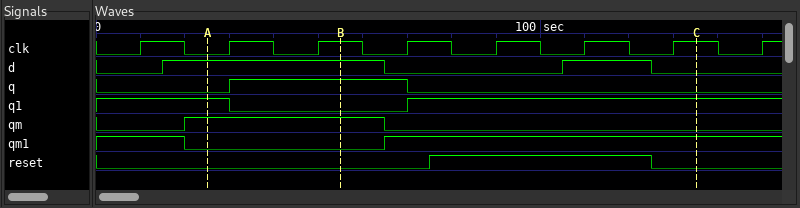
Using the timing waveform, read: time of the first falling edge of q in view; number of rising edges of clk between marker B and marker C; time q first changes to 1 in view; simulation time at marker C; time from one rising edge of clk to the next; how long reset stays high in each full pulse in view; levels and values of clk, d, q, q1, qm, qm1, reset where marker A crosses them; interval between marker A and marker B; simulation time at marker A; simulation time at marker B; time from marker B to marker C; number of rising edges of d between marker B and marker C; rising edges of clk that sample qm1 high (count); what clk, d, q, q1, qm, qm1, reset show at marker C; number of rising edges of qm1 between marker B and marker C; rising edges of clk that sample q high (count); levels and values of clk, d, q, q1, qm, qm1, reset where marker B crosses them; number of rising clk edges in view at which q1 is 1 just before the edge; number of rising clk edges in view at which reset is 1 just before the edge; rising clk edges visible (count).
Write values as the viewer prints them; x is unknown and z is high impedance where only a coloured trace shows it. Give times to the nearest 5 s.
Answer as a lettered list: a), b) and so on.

a) 70 s
b) 4
c) 30 s
d) 135 s
e) 20 s
f) 50 s
g) clk=0, d=1, q=0, q1=1, qm=1, qm1=0, reset=0
h) 30 s
i) 25 s
j) 55 s
k) 80 s
l) 1
m) 6
n) clk=1, d=0, q=0, q1=1, qm=0, qm1=1, reset=0
o) 1
p) 2
q) clk=1, d=1, q=1, q1=0, qm=1, qm1=0, reset=0
r) 6
s) 2
t) 8
